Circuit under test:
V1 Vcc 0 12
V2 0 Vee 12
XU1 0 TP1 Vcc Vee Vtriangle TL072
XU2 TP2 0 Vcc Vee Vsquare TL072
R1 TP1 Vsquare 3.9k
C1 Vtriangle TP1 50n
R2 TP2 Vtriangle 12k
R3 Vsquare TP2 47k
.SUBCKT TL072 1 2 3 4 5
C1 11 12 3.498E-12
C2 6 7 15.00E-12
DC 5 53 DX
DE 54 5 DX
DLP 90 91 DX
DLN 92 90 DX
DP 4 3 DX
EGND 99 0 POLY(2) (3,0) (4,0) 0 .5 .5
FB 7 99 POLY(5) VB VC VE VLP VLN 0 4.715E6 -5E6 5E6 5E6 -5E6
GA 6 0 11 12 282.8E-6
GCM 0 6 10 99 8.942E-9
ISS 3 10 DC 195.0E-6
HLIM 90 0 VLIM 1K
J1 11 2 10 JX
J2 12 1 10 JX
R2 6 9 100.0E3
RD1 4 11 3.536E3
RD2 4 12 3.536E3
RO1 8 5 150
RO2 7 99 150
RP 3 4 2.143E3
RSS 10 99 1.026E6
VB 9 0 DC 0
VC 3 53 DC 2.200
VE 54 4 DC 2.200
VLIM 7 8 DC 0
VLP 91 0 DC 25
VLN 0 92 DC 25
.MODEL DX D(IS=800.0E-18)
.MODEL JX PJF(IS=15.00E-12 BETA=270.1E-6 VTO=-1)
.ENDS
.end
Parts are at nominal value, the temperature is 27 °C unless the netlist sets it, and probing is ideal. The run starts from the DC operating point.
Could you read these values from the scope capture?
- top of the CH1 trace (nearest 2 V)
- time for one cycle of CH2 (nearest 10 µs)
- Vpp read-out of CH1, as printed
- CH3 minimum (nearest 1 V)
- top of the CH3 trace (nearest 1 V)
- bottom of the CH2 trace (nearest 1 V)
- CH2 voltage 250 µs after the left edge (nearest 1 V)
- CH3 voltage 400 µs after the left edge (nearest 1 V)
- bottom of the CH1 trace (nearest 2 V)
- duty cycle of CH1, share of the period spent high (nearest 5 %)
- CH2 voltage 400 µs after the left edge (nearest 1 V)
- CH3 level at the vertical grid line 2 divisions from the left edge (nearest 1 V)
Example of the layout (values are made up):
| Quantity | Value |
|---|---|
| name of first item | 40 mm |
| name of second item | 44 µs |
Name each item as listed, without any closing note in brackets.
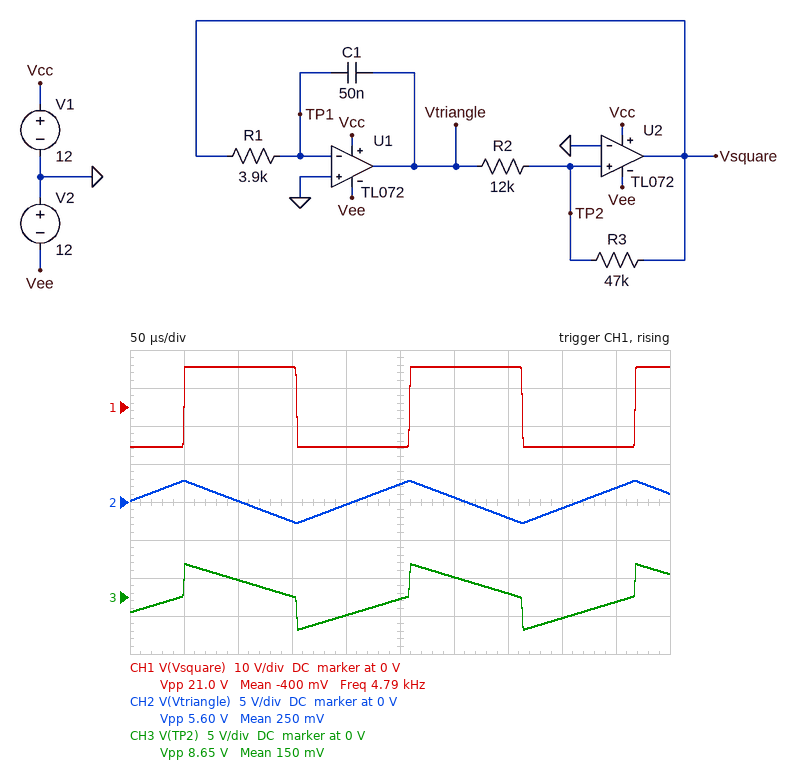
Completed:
| Quantity | Value |
|---|---|
| top of the CH1 trace | 10 V |
| time for one cycle of CH2 | 210 µs |
| Vpp read-out of CH1, as printed | 21.0 V |
| CH3 minimum | -4 V |
| top of the CH3 trace | 4 V |
| bottom of the CH2 trace | -3 V |
| CH2 voltage 250 µs after the left edge | 2 V |
| CH3 voltage 400 µs after the left edge | -3 V |
| bottom of the CH1 trace | -10 V |
| duty cycle of CH1, share of the period spent high | 50 % |
| CH2 voltage 400 µs after the left edge | -1 V |
| CH3 level at the vertical grid line 2 divisions from the left edge | 2 V |
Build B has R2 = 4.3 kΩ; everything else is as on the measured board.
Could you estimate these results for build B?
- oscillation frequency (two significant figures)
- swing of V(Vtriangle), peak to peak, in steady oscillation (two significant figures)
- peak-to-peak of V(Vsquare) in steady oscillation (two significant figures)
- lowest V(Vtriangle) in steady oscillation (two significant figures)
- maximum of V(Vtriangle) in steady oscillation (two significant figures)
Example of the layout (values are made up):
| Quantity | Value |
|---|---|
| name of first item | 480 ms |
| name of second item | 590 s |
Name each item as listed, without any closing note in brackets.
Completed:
| Quantity | Value |
|---|---|
| oscillation frequency | 12 kHz |
| swing of V(Vtriangle), peak to peak, in steady oscillation | 2.2 V |
| peak-to-peak of V(Vsquare) in steady oscillation | 21 V |
| lowest V(Vtriangle) in steady oscillation | -1.1 V |
| maximum of V(Vtriangle) in steady oscillation | 1.1 V |
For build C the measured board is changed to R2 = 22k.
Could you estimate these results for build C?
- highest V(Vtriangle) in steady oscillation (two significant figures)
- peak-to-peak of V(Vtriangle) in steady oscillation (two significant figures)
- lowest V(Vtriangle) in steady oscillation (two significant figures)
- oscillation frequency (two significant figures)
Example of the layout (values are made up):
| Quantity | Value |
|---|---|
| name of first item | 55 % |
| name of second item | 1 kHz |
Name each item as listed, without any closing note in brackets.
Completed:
| Quantity | Value |
|---|---|
| highest V(Vtriangle) in steady oscillation | 5.0 V |
| peak-to-peak of V(Vtriangle) in steady oscillation | 10 V |
| lowest V(Vtriangle) in steady oscillation | -5.0 V |
| oscillation frequency | 2.7 kHz |
